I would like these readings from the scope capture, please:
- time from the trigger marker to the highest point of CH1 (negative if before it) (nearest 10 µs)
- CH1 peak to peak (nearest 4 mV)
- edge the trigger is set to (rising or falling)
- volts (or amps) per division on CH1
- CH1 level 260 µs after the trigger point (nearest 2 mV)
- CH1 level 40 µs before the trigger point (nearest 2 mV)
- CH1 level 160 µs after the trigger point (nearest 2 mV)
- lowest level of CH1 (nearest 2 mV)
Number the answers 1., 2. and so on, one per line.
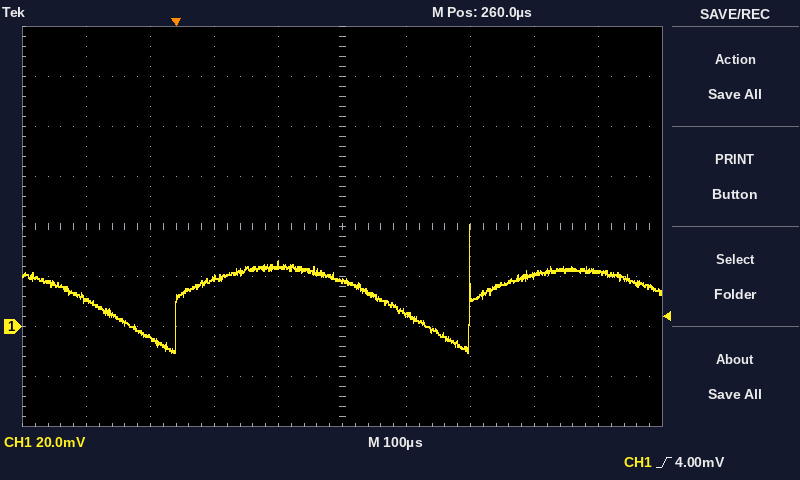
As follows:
1. +460 µs
2. 52 mV
3. rising
4. 20 mV
5. 18 mV
6. -4 mV
7. 24 mV
8. -10 mV
